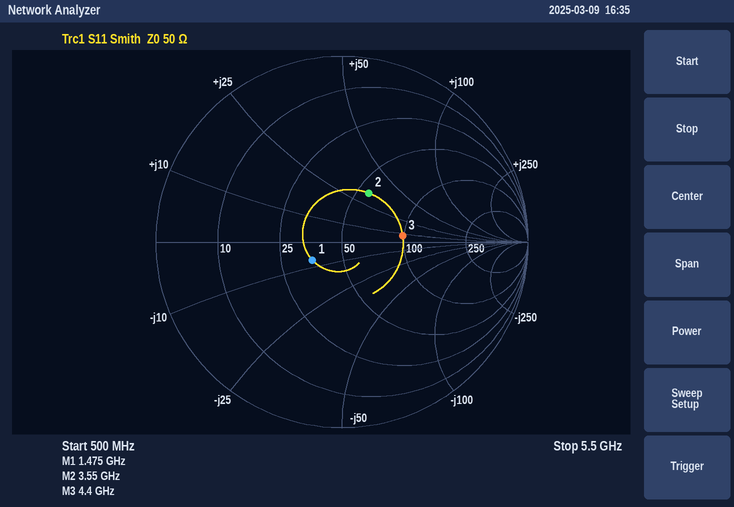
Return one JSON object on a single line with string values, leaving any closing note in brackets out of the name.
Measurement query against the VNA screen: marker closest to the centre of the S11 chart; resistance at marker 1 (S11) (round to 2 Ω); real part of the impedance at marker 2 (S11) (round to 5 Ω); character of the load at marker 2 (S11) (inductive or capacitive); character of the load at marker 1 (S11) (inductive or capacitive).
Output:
{"marker closest to the centre of the S11 chart": "marker 1", "resistance at marker 1 (S11)": "36 Ω", "real part of the impedance at marker 2 (S11)": "55 Ω", "character of the load at marker 2 (S11)": "inductive", "character of the load at marker 1 (S11)": "capacitive"}
